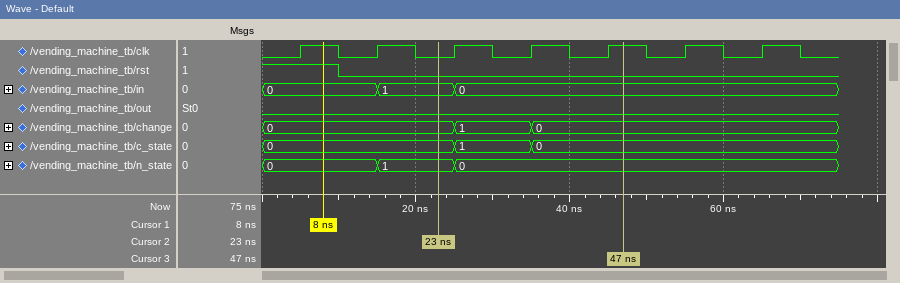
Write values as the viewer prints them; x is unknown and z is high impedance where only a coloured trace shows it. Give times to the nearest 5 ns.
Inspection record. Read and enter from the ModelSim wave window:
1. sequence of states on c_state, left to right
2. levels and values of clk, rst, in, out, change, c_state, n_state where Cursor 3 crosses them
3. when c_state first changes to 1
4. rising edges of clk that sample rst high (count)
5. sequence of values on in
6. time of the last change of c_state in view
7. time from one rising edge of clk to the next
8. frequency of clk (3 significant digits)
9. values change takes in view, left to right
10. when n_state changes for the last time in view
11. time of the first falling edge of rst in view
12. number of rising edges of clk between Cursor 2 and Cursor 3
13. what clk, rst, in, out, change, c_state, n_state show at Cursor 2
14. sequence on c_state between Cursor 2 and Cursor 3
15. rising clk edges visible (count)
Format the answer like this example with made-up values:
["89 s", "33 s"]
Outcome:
["0, 1, 0", "clk=1, rst=0, in=0, out=0, change=0, c_state=0, n_state=0", "25 ns", "1", "0, 1, 0", "35 ns", "10 ns", "100 MHz", "0, 1, 0", "25 ns", "10 ns", "3", "clk=0, rst=0, in=1, out=0, change=0, c_state=0, n_state=1", "0, 1, 0", "7"]
